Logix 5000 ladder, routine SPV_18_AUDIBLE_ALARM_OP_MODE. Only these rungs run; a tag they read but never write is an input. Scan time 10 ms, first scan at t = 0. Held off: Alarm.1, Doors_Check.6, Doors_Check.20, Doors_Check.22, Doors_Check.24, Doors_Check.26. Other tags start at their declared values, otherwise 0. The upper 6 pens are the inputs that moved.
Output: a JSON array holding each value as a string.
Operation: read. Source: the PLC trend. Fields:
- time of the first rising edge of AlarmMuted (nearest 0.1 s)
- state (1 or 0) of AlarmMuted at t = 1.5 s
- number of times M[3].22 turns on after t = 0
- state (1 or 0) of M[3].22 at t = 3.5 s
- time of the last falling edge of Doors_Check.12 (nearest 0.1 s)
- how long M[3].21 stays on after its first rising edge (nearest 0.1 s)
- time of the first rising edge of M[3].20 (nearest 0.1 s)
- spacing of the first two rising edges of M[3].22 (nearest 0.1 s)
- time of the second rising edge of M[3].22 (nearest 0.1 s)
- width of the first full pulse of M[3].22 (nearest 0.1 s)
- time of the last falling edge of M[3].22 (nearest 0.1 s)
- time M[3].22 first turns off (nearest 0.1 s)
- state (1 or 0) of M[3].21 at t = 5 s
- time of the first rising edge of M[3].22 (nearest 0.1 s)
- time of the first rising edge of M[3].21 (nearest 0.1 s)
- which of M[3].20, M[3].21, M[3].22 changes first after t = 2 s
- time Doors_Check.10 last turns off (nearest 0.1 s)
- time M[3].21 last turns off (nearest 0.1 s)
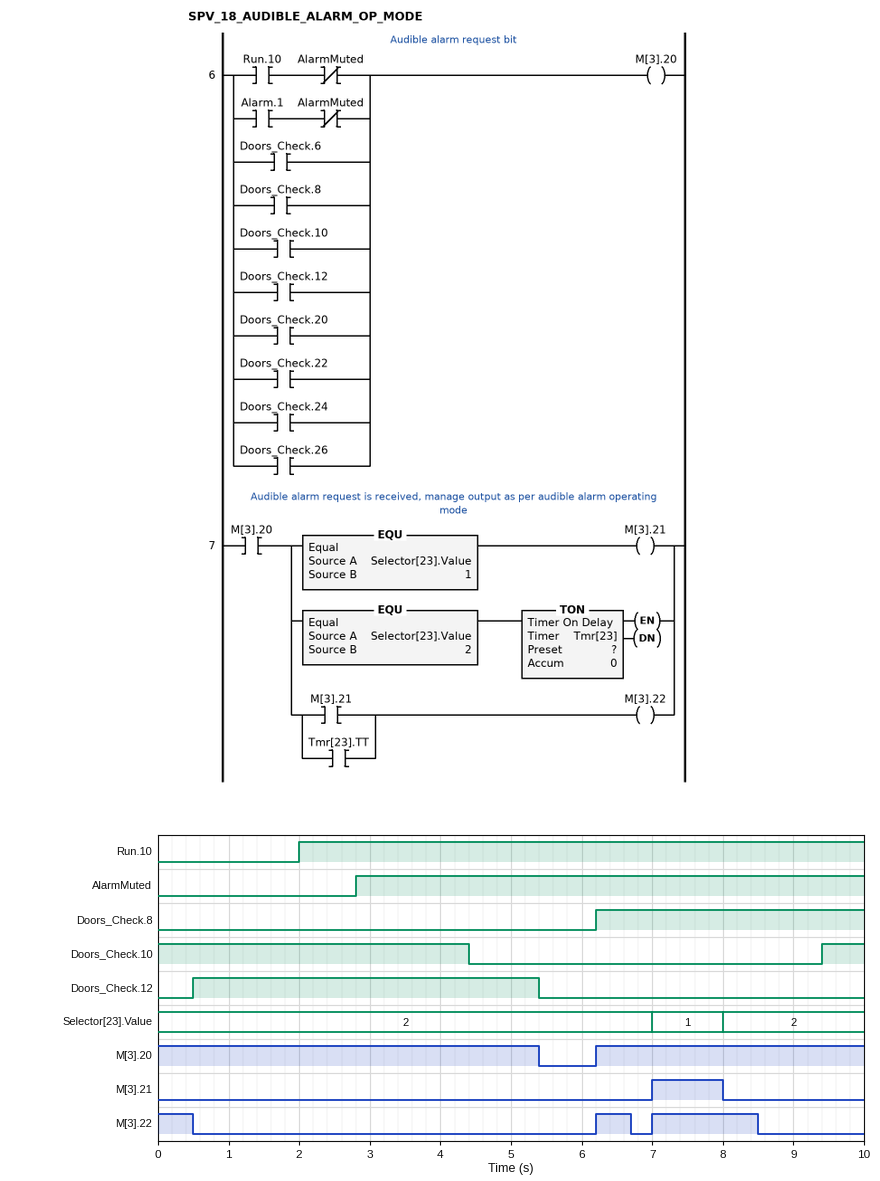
["2.8 s", "0", "2", "0", "5.4 s", "1.0 s", "6.2 s", "0.8 s", "7.0 s", "0.5 s", "8.5 s", "0.5 s", "0", "6.2 s", "7.0 s", "M[3].20", "4.4 s", "8.0 s"]
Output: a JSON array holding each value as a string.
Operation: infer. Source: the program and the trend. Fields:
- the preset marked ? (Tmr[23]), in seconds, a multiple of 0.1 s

["0.5 s"]
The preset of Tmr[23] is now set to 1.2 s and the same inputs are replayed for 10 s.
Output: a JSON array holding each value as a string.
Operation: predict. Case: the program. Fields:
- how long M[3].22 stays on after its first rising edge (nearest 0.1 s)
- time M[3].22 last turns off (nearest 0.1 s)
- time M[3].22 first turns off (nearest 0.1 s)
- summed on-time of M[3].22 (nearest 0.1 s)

["3.0 s", "9.2 s", "1.2 s", "4.2 s"]
